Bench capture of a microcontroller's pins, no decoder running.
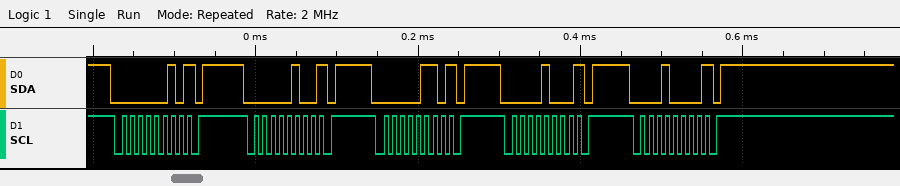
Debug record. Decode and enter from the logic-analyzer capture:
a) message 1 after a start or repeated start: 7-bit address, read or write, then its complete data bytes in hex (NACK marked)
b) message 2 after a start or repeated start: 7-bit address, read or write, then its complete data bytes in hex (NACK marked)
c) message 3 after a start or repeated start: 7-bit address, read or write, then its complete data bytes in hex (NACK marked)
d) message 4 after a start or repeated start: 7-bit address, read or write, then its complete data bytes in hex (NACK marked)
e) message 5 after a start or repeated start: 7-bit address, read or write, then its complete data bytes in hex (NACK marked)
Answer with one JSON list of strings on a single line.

["0x01 write NACK", "0x02 write NACK", "0x03 write NACK", "0x04 write NACK", "0x08 write NACK"]
